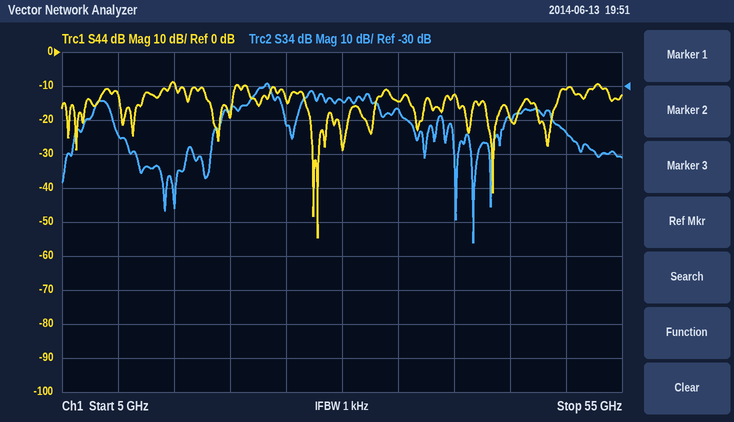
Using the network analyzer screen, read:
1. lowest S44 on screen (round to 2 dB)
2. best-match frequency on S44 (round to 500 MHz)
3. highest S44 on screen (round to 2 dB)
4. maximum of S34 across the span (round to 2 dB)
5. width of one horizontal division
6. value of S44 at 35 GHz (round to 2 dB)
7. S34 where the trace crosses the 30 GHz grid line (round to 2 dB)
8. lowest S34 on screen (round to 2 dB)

-54 dB
28.0 GHz
-8 dB
-30 dB
5 GHz
-14 dB
-34 dB
-76 dB
